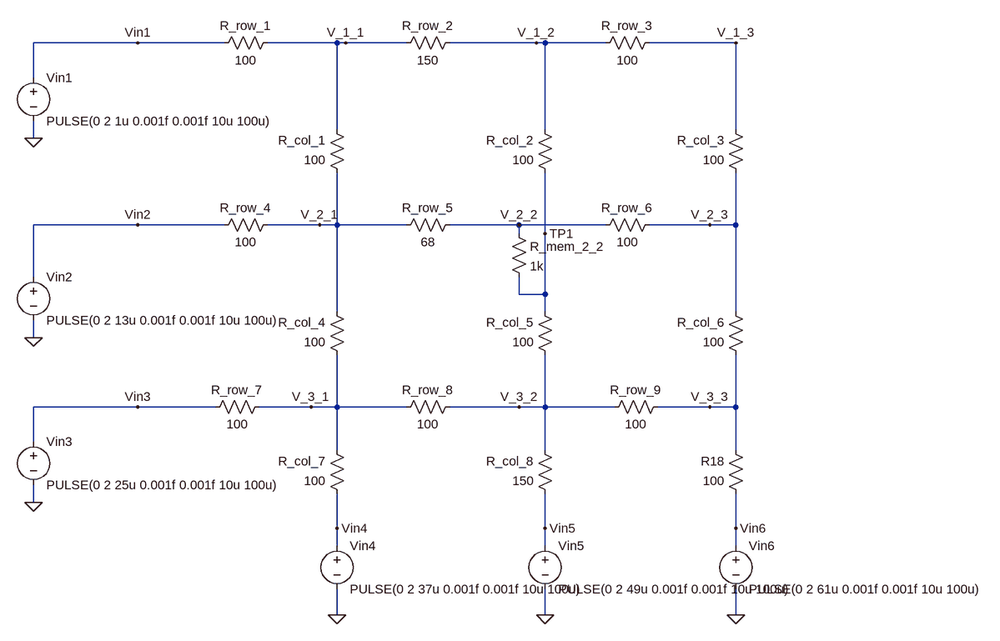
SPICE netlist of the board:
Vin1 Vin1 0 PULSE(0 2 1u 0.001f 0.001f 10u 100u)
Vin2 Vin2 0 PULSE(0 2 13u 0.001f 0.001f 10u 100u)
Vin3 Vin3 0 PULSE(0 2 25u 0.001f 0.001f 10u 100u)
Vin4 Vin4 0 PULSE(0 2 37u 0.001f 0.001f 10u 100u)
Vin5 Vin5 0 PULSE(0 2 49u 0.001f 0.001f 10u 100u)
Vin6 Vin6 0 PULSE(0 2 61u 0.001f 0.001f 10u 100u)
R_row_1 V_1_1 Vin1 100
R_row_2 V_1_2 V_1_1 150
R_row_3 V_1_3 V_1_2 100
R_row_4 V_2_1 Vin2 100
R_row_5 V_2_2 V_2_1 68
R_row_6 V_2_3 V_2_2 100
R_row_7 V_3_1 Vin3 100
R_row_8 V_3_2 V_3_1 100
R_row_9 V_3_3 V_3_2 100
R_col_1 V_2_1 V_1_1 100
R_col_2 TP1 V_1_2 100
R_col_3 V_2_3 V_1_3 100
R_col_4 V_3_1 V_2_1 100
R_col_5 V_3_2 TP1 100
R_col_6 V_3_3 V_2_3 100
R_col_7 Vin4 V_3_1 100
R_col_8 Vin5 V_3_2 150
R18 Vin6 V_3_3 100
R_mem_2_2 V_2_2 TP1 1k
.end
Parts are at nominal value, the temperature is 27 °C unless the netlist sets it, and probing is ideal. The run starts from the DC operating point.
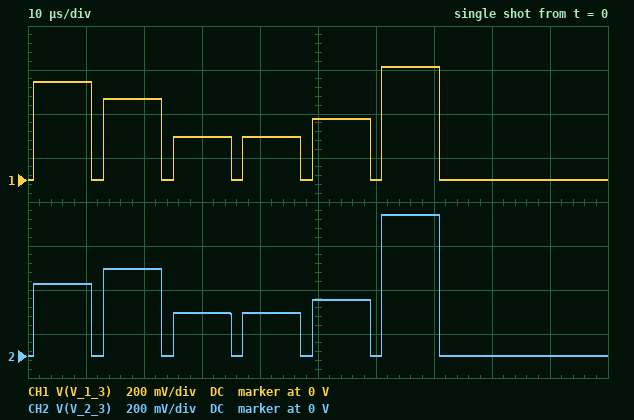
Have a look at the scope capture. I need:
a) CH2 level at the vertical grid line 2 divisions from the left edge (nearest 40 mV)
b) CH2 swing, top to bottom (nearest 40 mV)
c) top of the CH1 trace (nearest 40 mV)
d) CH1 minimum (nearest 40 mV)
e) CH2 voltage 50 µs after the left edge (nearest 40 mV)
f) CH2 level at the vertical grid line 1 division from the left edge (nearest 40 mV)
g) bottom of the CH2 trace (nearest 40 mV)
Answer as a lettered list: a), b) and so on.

a) 400 mV
b) 640 mV
c) 520 mV
d) 0 V
e) 240 mV
f) 320 mV
g) 0 V
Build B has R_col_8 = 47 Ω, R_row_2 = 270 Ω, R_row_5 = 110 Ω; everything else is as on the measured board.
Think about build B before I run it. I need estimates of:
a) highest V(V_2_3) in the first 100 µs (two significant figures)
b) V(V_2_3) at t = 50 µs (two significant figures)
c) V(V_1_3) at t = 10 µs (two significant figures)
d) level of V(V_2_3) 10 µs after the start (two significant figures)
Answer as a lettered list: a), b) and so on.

a) 610 mV
b) 530 mV
c) 340 mV
d) 250 mV
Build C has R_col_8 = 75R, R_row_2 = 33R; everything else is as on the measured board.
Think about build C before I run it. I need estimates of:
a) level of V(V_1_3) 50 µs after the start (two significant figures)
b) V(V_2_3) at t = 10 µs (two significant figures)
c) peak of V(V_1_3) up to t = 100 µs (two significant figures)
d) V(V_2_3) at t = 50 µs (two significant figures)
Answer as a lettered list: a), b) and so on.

a) 340 mV
b) 380 mV
c) 570 mV
d) 350 mV
